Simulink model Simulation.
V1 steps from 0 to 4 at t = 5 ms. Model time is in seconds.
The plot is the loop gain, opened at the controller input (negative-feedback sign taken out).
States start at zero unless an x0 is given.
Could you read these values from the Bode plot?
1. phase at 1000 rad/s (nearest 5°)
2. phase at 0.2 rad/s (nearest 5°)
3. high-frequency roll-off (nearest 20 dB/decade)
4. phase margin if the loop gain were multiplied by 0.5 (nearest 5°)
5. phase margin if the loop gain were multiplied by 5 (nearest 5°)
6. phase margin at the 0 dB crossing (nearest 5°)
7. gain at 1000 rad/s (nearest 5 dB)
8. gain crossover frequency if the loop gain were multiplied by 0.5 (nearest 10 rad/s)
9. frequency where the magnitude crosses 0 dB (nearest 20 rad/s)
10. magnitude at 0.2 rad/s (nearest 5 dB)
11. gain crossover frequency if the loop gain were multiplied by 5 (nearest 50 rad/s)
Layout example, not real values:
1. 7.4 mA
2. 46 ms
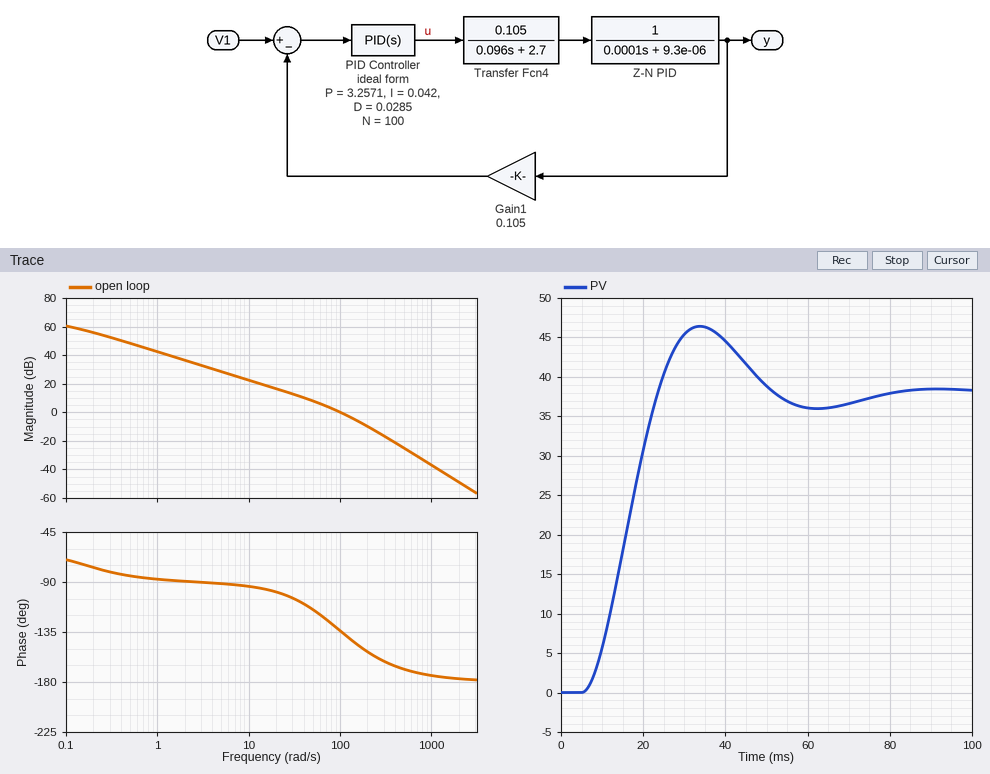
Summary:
1. -175°
2. -75°
3. -40 dB/decade
4. 60°
5. 20°
6. 45°
7. -35 dB
8. 60 rad/s
9. 100 rad/s
10. 55 dB
11. 250 rad/s
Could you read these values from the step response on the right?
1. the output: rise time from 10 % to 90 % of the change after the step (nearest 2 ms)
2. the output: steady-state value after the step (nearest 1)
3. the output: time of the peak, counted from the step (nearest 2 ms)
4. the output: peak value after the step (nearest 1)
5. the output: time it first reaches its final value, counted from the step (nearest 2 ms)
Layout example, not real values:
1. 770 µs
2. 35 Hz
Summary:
1. 12 ms
2. 38
3. 28 ms
4. 46
5. 18 ms
